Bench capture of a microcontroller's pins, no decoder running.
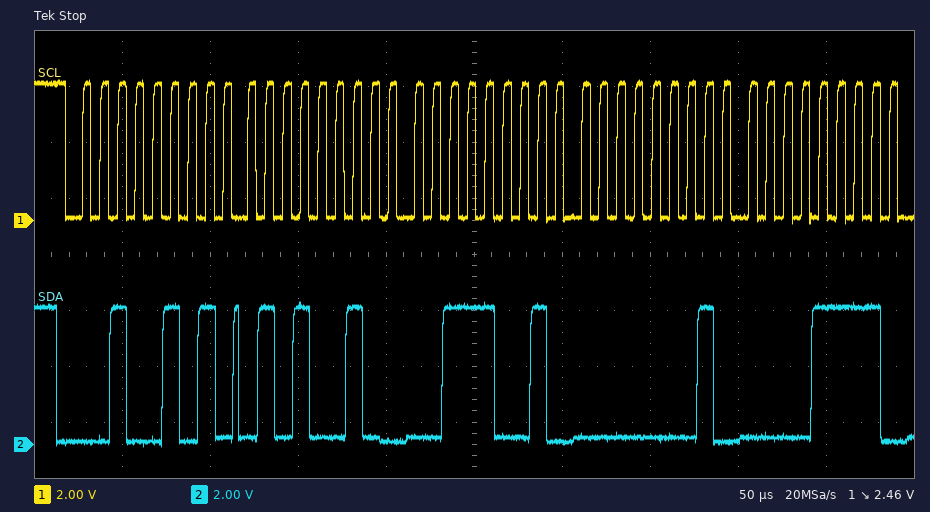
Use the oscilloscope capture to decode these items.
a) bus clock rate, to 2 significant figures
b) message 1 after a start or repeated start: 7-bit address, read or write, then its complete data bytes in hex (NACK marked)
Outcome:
100 kHz
0x12 read: 52 39 01 0F
